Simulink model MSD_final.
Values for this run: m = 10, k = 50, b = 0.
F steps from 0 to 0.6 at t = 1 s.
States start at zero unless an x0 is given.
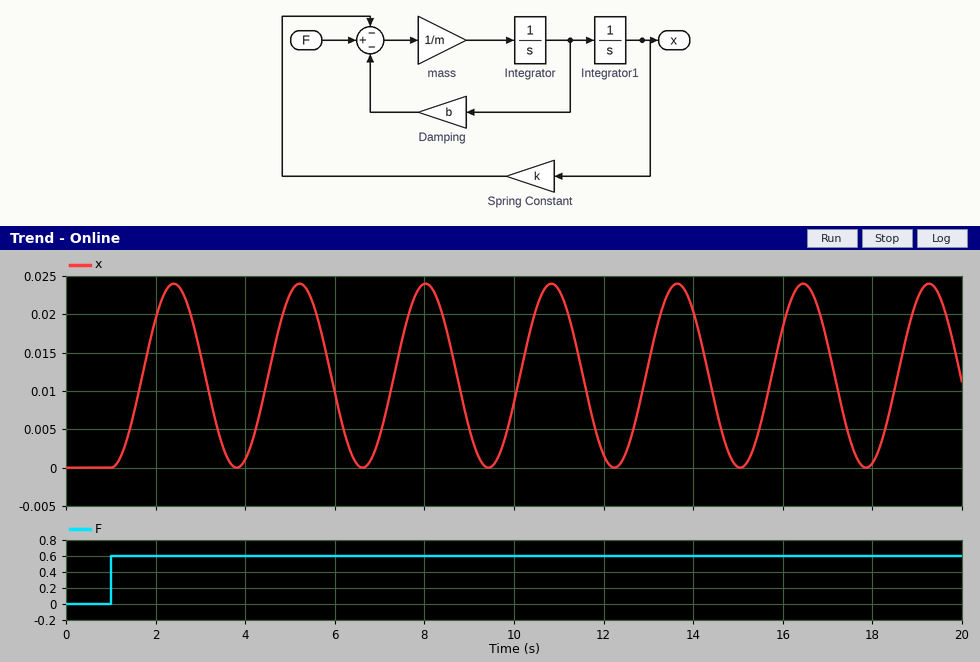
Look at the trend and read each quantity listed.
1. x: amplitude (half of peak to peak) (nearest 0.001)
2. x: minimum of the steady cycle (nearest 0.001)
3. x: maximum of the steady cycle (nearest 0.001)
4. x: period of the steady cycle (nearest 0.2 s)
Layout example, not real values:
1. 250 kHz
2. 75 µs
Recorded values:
1. 0.012
2. 0.000
3. 0.024
4. 2.8 s
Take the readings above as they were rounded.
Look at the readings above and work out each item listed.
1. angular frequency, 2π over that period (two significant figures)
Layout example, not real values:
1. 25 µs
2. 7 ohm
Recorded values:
1. 2.2 rad/s
